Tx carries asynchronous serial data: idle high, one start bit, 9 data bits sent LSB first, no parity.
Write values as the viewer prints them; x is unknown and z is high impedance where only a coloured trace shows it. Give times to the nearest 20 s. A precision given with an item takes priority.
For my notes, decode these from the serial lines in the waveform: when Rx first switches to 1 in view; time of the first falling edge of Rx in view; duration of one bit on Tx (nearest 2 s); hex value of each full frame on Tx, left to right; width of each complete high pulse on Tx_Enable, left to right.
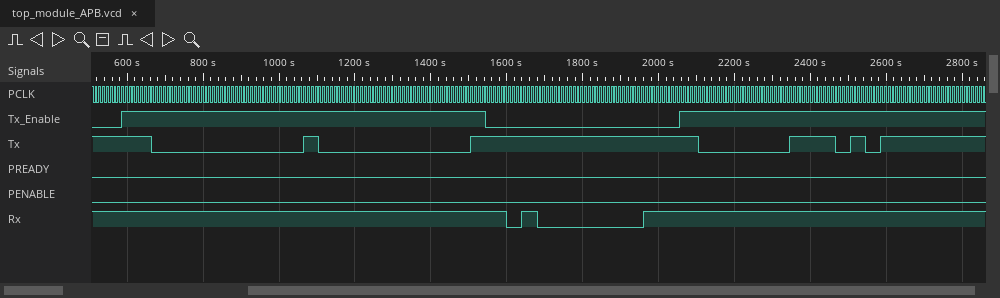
1640 s
1600 s
40 s
00, 00, E0
960 s
